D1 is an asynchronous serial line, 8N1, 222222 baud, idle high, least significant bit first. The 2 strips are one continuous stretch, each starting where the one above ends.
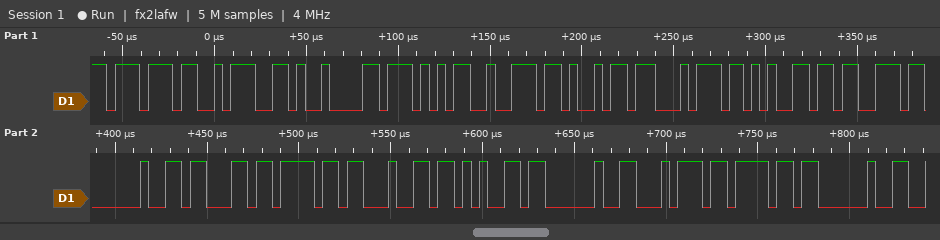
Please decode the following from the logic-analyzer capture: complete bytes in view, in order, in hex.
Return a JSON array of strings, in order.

["77 3A 09 57 72 69 74 65 73 20 63 6F 64 65 20 74 6F 20"]
